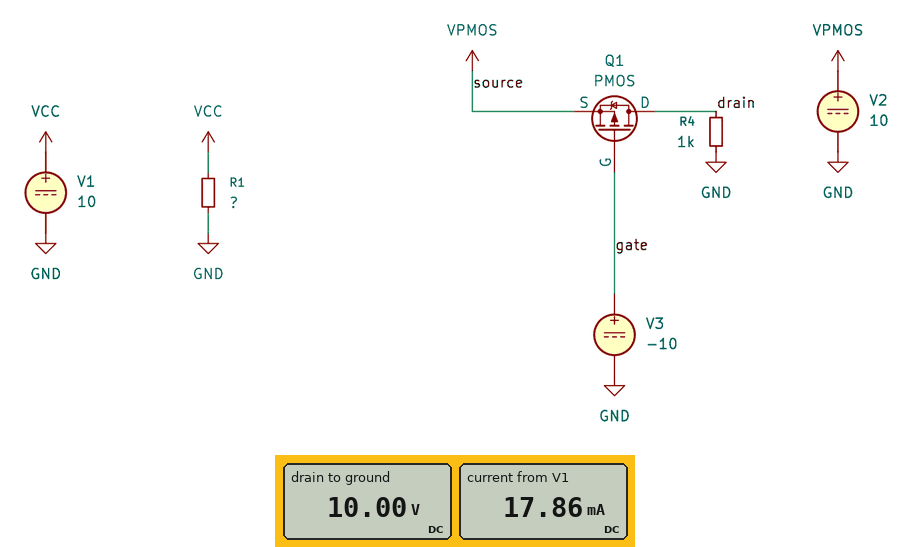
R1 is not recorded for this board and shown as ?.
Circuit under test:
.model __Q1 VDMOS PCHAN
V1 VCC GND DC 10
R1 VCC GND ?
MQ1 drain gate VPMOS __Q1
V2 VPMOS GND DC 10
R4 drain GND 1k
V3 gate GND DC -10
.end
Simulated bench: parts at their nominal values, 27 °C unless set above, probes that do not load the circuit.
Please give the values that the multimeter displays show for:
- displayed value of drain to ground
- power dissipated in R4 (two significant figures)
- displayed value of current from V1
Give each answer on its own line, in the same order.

10.00 V
100 mW
17.86 mA
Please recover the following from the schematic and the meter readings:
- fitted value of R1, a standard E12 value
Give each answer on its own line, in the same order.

560 Ω
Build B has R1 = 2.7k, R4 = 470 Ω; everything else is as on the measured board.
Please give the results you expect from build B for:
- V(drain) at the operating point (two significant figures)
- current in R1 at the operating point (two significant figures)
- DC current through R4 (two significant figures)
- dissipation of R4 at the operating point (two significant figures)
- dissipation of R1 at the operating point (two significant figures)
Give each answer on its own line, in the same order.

10 V
3.7 mA
21 mA
210 mW
37 mW
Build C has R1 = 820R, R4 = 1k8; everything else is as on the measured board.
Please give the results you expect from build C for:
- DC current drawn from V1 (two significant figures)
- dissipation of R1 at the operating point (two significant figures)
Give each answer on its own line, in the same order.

12 mA
120 mW
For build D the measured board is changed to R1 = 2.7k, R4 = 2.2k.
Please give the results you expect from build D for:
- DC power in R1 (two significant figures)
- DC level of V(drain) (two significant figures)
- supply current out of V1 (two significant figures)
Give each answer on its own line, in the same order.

37 mW
10 V
3.7 mA
